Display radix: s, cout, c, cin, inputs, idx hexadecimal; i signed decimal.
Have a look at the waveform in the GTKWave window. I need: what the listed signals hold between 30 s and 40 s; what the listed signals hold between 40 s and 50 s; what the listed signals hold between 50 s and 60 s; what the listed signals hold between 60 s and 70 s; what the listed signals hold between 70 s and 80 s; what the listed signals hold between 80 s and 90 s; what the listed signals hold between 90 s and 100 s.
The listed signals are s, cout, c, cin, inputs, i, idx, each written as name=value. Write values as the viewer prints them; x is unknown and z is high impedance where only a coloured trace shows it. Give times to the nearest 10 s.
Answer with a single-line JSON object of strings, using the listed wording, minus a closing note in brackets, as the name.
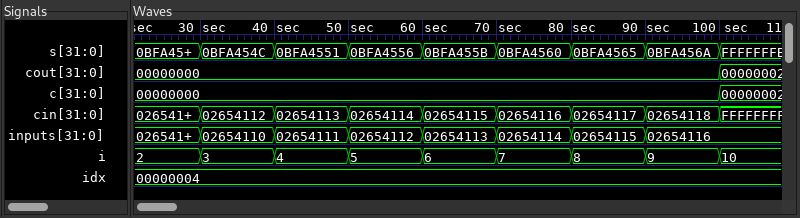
{"what the listed signals hold between 30 s and 40 s": "s=0BFA454C, cout=00000000, c=00000000, cin=02654112, inputs=02654110, i=3, idx=00000004", "what the listed signals hold between 40 s and 50 s": "s=0BFA4551, cout=00000000, c=00000000, cin=02654113, inputs=02654111, i=4, idx=00000004", "what the listed signals hold between 50 s and 60 s": "s=0BFA4556, cout=00000000, c=00000000, cin=02654114, inputs=02654112, i=5, idx=00000004", "what the listed signals hold between 60 s and 70 s": "s=0BFA455B, cout=00000000, c=00000000, cin=02654115, inputs=02654113, i=6, idx=00000004", "what the listed signals hold between 70 s and 80 s": "s=0BFA4560, cout=00000000, c=00000000, cin=02654116, inputs=02654114, i=7, idx=00000004", "what the listed signals hold between 80 s and 90 s": "s=0BFA4565, cout=00000000, c=00000000, cin=02654117, inputs=02654115, i=8, idx=00000004", "what the listed signals hold between 90 s and 100 s": "s=0BFA456A, cout=00000000, c=00000000, cin=02654118, inputs=02654116, i=9, idx=00000004"}
